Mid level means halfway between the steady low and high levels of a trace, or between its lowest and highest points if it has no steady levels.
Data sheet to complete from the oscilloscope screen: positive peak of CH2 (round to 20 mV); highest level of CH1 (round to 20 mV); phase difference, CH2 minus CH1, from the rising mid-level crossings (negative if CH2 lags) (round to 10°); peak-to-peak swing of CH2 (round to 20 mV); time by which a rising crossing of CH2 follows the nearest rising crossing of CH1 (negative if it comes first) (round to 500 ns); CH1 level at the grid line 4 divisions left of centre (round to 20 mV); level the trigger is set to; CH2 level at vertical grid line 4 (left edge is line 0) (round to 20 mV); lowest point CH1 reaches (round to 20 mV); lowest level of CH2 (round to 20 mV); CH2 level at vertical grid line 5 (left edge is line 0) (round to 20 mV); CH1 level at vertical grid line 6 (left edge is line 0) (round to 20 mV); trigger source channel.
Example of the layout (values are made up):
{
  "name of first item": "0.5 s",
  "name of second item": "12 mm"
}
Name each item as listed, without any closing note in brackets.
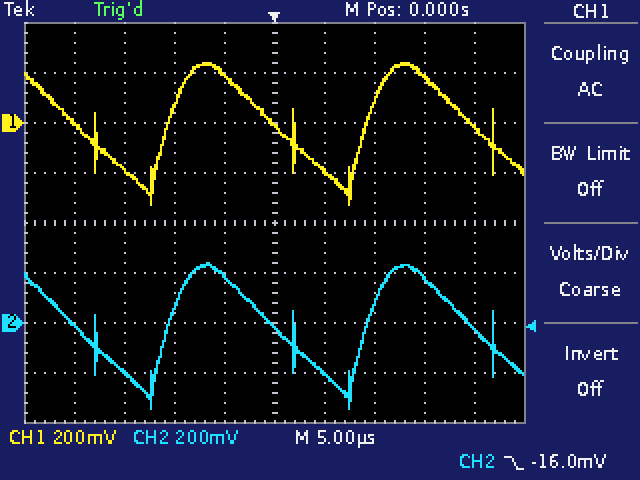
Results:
{
  "positive peak of CH2": "240 mV",
  "highest level of CH1": "240 mV",
  "phase difference, CH2 minus CH1, from the rising mid-level crossings (negative if CH2 lags)": "0°",
  "peak-to-peak swing of CH2": "580 mV",
  "time by which a rising crossing of CH2 follows the nearest rising crossing of CH1 (negative if it comes first)": "0.0 µs",
  "CH1 level at the grid line 4 divisions left of centre": "0 mV",
  "level the trigger is set to": "-16.0 mV",
  "CH2 level at vertical grid line 4 (left edge is line 0)": "180 mV",
  "lowest point CH1 reaches": "-320 mV",
  "lowest level of CH2": "-340 mV",
  "CH2 level at vertical grid line 5 (left edge is line 0)": "-20 mV",
  "CH1 level at vertical grid line 6 (left edge is line 0)": "-200 mV",
  "trigger source channel": "CH2"
}
